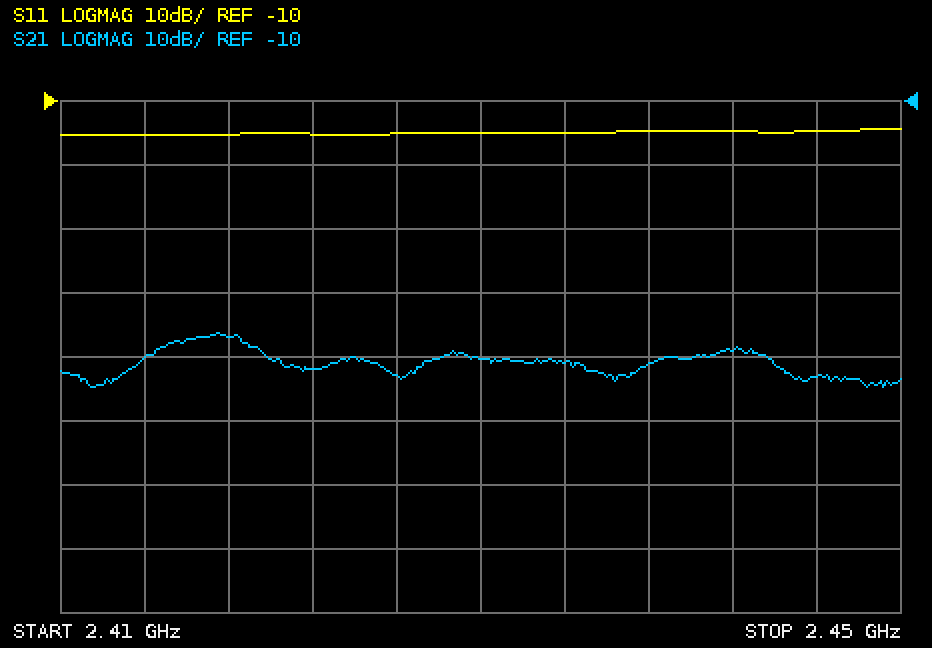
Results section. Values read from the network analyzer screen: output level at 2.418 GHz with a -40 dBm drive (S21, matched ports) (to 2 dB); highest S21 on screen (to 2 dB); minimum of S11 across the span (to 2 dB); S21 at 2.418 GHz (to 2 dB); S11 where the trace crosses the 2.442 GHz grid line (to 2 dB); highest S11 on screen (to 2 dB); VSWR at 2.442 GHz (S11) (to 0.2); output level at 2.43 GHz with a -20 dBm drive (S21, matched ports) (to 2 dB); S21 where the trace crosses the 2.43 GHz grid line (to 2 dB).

-86 dBm
-46 dB
-16 dB
-46 dB
-14 dB
-14 dB
1.4
-70 dBm
-50 dB
